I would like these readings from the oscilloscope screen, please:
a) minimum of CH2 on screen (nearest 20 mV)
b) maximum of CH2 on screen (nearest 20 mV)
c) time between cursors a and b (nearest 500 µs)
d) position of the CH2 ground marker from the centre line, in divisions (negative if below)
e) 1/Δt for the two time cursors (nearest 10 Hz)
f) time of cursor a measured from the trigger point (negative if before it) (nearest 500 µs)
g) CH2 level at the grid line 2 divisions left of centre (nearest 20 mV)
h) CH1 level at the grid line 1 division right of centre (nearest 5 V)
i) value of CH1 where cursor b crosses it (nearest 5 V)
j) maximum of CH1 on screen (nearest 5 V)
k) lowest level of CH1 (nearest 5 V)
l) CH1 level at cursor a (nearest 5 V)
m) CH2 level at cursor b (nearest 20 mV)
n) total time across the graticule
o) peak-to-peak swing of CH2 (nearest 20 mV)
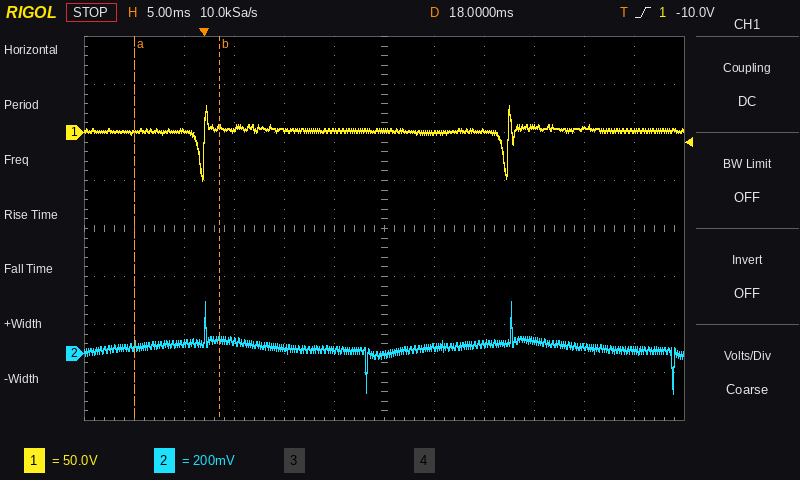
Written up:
-160 mV
220 mV
8.5 ms
-2.6 div
120 Hz
-7.0 ms
20 mV
0 V
5 V
30 V
-50 V
0 V
60 mV
60 ms
380 mV
